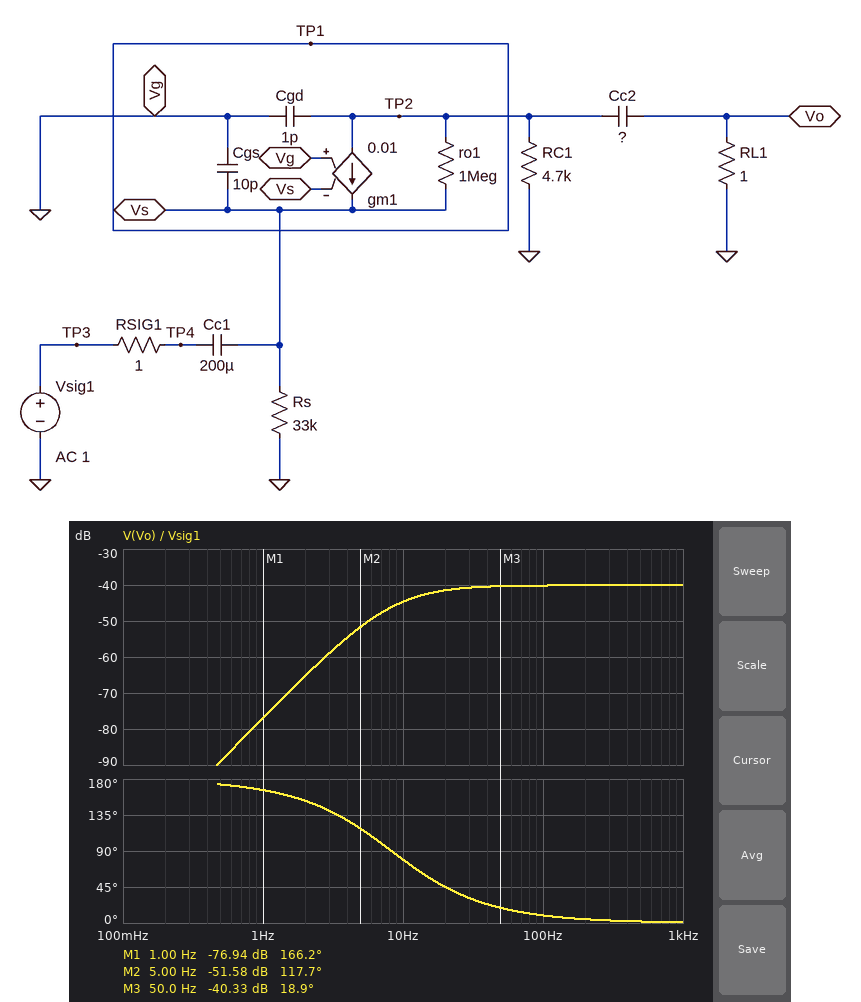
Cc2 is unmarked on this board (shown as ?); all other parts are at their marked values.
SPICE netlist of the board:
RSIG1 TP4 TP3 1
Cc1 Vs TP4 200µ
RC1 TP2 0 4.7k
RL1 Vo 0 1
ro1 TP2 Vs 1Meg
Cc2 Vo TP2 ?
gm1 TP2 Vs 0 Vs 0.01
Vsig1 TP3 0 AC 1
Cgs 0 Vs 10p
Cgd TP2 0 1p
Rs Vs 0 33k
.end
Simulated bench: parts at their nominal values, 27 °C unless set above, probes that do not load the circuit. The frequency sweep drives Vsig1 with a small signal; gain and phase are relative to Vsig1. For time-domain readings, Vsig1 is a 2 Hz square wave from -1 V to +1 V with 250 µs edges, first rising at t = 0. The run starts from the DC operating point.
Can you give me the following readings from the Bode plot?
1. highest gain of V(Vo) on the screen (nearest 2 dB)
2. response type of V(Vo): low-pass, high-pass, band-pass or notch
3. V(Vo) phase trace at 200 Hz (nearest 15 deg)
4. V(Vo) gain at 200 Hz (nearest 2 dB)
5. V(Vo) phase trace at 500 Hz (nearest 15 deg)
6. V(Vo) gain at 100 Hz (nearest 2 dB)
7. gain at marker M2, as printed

-40 dB
high-pass
0 deg
-40 dB
0 deg
-40 dB
-51.58 dB
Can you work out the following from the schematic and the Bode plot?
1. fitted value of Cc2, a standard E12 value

3.9 µF
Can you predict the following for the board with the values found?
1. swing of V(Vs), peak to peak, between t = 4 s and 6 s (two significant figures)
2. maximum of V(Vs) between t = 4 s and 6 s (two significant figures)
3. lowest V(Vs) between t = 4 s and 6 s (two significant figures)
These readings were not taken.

3.9 V
2.0 V
-2.0 V
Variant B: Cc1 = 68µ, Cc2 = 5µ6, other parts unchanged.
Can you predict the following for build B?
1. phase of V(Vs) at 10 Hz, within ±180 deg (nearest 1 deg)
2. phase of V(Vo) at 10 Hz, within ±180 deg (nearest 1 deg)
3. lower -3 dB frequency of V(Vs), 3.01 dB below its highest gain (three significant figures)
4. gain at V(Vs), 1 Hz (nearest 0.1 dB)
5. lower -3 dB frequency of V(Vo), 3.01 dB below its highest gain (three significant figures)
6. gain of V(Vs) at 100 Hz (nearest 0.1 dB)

67 deg
98 deg
23.3 Hz
-27.4 dB
24.7 Hz
-0.3 dB
